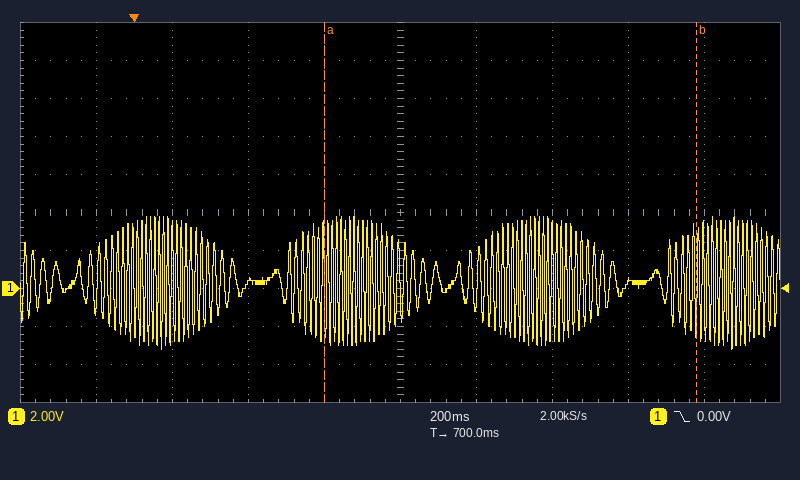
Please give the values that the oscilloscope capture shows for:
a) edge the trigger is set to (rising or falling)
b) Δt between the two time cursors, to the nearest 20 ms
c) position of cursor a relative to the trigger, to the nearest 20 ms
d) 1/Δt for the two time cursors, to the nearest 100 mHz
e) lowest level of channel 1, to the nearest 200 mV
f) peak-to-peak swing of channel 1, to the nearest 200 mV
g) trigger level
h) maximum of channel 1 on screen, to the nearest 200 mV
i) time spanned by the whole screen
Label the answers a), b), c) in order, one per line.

a) falling
b) 980 ms
c) +500 ms
d) 1.0 Hz
e) -3.2 V
f) 7.0 V
g) 0.00 V
h) 3.8 V
i) 2 s
